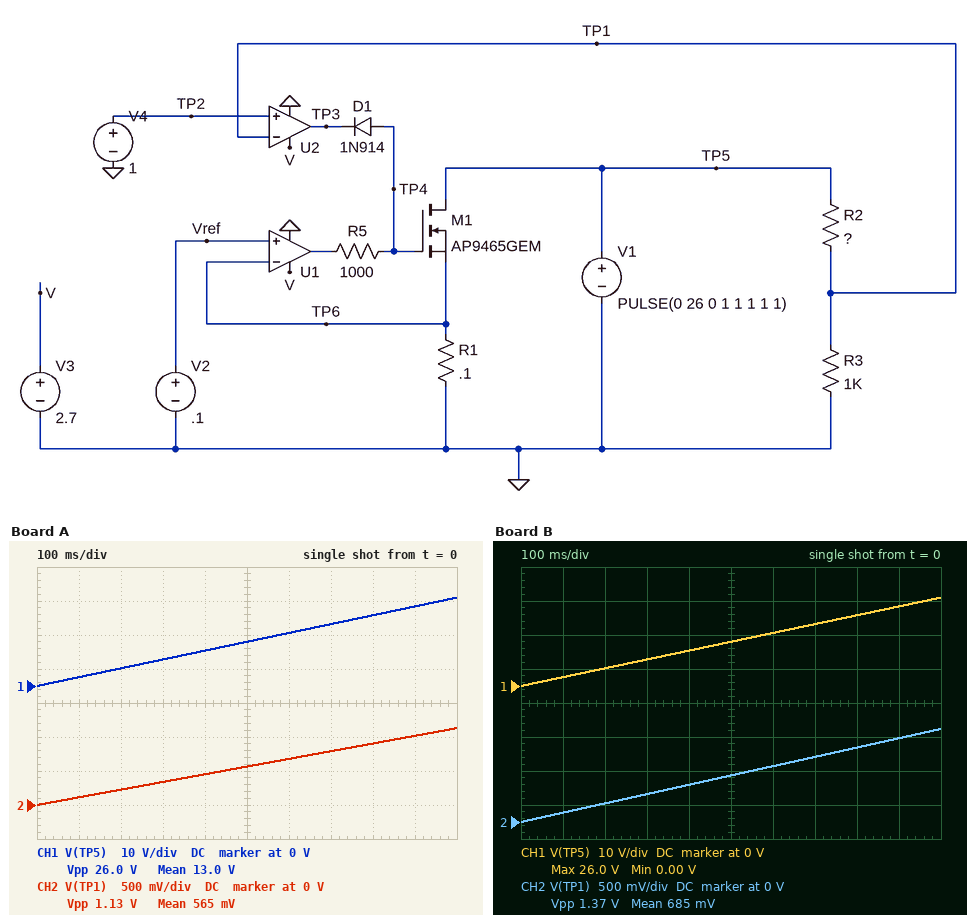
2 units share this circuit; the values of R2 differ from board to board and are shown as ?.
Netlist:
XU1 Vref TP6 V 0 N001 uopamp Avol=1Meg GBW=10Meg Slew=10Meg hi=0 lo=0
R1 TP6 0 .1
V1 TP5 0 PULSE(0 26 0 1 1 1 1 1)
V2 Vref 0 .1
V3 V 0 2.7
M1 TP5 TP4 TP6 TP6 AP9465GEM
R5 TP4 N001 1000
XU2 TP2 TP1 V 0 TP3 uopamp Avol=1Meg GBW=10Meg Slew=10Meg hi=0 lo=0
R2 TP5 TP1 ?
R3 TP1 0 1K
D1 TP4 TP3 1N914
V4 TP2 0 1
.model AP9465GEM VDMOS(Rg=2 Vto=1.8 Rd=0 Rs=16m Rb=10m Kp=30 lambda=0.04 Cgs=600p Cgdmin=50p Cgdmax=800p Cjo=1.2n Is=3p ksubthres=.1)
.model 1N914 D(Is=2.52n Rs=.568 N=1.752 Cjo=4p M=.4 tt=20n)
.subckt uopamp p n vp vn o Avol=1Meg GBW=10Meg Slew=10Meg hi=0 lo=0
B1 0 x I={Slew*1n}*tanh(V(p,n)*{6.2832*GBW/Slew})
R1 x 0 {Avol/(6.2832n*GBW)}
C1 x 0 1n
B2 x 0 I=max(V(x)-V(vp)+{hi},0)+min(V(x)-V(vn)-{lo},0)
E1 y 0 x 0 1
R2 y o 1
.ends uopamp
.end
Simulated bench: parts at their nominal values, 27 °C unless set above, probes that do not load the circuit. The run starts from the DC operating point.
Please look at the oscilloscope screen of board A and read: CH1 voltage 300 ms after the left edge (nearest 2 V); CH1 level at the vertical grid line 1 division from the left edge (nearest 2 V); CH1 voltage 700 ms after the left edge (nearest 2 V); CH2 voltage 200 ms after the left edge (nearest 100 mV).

8 V
2 V
18 V
200 mV
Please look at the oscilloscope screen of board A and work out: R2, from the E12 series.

22 kΩ
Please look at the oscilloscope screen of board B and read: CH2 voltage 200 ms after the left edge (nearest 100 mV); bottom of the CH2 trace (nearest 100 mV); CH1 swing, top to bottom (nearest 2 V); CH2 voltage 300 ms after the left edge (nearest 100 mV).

300 mV
0 V
26 V
400 mV
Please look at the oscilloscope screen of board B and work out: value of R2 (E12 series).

18 kΩ
